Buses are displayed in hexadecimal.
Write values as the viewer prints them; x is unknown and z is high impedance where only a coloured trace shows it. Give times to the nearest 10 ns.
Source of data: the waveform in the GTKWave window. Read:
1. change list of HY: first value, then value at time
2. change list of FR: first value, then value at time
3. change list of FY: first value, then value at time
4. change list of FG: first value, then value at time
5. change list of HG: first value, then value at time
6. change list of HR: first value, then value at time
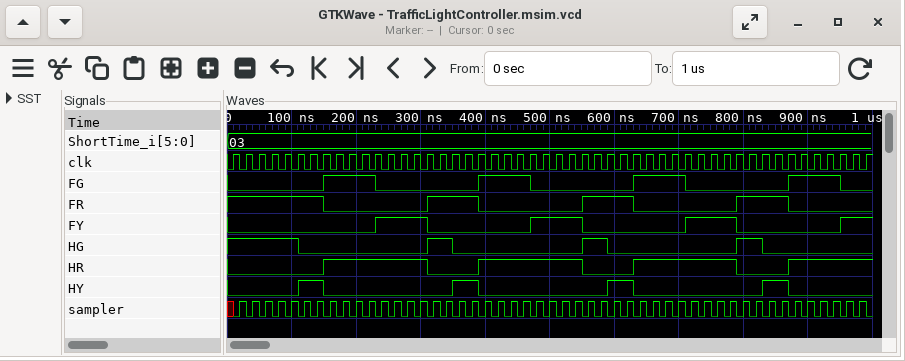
0, 1 at 110 ns, 0 at 150 ns, 1 at 350 ns, 0 at 390 ns, 1 at 590 ns, 0 at 630 ns, 1 at 830 ns, 0 at 870 ns
1, 0 at 150 ns, 1 at 310 ns, 0 at 390 ns, 1 at 550 ns, 0 at 630 ns, 1 at 790 ns, 0 at 870 ns
0, 1 at 230 ns, 0 at 310 ns, 1 at 470 ns, 0 at 550 ns, 1 at 710 ns, 0 at 790 ns, 1 at 950 ns
0, 1 at 150 ns, 0 at 230 ns, 1 at 390 ns, 0 at 470 ns, 1 at 630 ns, 0 at 710 ns, 1 at 870 ns, 0 at 950 ns
1, 0 at 110 ns, 1 at 310 ns, 0 at 350 ns, 1 at 550 ns, 0 at 590 ns, 1 at 790 ns, 0 at 830 ns
0, 1 at 150 ns, 0 at 310 ns, 1 at 390 ns, 0 at 550 ns, 1 at 630 ns, 0 at 790 ns, 1 at 870 ns
